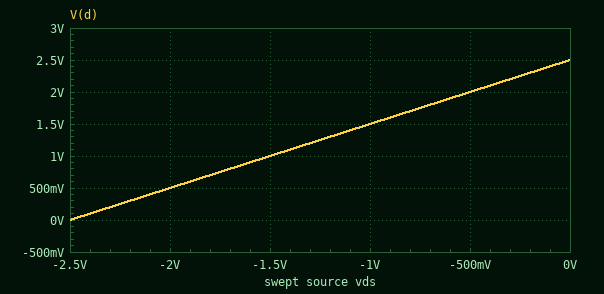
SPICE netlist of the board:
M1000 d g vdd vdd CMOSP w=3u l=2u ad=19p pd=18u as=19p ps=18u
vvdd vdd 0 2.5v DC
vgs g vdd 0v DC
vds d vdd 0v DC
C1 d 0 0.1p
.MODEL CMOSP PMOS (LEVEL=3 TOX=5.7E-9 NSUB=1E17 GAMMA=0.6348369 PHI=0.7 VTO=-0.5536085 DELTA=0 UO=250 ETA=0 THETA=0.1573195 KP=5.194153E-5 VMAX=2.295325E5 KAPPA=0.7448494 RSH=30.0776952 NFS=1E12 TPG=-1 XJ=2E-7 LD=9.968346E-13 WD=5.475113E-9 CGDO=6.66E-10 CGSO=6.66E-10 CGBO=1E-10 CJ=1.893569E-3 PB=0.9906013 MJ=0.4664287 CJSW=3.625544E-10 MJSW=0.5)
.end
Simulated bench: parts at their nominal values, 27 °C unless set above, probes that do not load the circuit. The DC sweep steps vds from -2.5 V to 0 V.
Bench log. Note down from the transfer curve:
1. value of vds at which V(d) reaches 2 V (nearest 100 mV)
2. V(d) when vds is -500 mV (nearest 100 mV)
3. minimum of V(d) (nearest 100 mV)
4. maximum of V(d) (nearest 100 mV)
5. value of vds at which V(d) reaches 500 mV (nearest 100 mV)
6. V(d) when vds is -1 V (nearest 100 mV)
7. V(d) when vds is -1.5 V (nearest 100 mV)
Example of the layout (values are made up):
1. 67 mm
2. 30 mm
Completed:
1. -500 mV
2. 2.0 V
3. 0 V
4. 2.5 V
5. -2.0 V
6. 1.5 V
7. 1.0 V
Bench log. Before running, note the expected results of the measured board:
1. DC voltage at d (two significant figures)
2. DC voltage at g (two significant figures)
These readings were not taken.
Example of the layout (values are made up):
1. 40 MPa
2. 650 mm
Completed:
1. 2.5 V
2. 2.5 V
